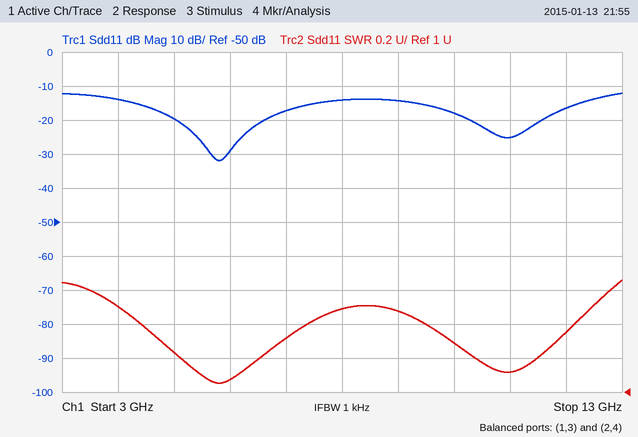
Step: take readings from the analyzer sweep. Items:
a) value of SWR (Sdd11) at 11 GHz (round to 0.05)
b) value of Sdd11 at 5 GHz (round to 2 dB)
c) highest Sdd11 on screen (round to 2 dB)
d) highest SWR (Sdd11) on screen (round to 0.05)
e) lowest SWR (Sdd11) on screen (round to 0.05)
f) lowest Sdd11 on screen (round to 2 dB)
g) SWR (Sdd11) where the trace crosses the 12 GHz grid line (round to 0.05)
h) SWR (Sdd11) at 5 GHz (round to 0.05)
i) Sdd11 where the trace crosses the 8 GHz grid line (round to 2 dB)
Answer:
1.10
-20 dB
-12 dB
1.65
1.05
-32 dB
1.35
1.25
-14 dB
